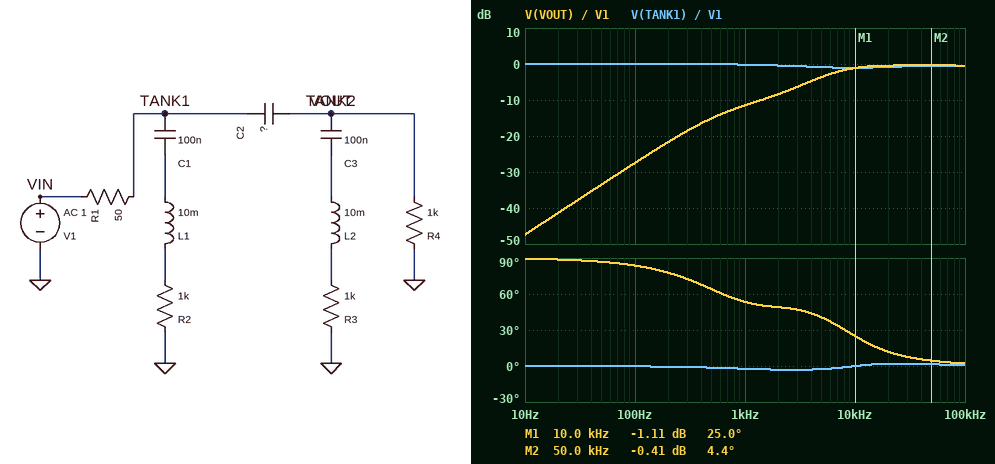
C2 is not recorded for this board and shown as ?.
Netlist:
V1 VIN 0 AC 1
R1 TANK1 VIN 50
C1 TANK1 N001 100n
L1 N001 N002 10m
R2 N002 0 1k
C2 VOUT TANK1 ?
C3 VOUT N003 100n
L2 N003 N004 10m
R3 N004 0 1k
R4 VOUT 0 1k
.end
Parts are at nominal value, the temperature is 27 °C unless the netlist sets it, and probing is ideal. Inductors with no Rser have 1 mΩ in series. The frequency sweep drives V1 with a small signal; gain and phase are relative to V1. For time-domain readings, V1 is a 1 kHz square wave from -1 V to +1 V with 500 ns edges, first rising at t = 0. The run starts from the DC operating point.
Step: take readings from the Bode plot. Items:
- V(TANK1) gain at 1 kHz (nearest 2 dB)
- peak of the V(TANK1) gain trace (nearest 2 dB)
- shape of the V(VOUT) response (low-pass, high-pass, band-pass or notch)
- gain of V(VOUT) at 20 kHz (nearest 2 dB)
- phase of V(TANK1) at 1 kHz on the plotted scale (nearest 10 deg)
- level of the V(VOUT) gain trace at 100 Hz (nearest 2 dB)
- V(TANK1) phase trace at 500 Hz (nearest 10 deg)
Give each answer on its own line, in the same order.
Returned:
0 dB
0 dB
high-pass
0 dB
0 deg
-28 dB
0 deg
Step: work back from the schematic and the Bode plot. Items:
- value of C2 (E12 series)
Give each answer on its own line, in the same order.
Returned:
68 nF
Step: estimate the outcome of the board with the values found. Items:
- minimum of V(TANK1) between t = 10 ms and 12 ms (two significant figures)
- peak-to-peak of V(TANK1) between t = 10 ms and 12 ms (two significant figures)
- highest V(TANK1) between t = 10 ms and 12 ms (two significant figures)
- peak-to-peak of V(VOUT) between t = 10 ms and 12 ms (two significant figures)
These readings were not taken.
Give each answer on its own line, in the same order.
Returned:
-1.0 V
2.0 V
1.0 V
3.7 V
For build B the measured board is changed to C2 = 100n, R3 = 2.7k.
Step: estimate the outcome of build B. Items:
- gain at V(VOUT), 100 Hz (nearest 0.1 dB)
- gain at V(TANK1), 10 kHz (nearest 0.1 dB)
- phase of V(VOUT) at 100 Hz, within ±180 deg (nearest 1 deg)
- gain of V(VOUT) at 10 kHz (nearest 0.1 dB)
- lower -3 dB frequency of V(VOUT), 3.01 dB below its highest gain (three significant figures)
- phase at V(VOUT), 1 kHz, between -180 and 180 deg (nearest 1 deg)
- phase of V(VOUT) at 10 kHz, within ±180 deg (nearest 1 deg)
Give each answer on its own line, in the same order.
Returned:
-24.2 dB
-0.9 dB
83 deg
-1.0 dB
2.40 kHz
56 deg
13 deg
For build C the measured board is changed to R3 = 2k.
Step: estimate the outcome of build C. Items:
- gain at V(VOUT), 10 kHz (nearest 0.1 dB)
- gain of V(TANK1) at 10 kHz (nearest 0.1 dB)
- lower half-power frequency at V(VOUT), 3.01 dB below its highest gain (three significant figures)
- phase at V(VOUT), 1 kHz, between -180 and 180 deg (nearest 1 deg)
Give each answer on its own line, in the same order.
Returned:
-1.2 dB
-0.9 dB
3.90 kHz
61 deg
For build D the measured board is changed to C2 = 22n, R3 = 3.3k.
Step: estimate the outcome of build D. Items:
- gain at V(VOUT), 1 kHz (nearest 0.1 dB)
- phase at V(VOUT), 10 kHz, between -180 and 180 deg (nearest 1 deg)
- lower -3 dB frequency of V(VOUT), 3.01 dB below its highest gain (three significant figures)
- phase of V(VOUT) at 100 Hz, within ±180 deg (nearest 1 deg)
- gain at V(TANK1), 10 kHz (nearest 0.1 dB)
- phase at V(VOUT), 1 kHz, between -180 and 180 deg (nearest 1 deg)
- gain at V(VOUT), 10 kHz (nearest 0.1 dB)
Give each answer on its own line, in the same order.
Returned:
-19.4 dB
43 deg
9.59 kHz
86 deg
-0.6 dB
77 deg
-3.2 dB
